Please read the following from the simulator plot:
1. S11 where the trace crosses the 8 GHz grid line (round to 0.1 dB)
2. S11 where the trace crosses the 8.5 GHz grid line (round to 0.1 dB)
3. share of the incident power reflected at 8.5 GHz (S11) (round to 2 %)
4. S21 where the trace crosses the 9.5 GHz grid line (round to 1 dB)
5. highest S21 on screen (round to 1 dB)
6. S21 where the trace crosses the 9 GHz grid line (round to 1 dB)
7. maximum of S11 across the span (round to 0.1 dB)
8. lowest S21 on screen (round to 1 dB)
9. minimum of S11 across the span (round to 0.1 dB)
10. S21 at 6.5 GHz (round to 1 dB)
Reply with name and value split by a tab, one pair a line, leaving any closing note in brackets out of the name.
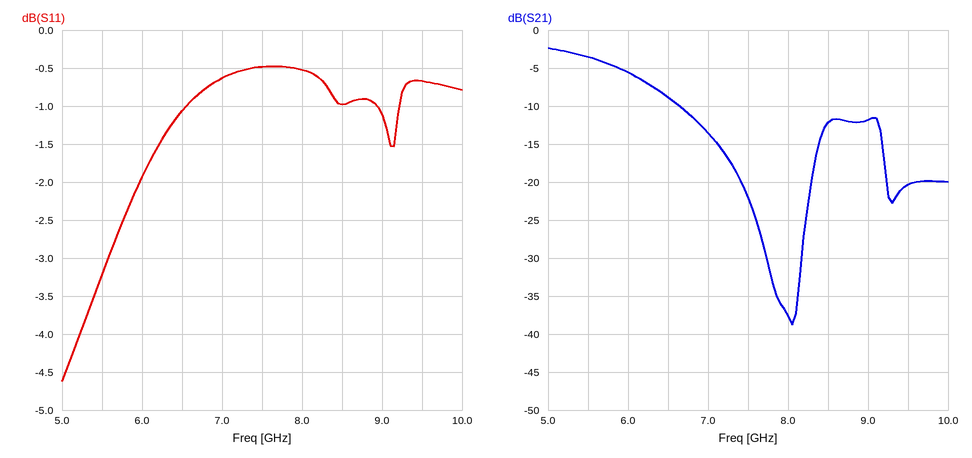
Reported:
S11 where the trace crosses the 8 GHz grid line	-0.5 dB
S11 where the trace crosses the 8.5 GHz grid line	-1.0 dB
share of the incident power reflected at 8.5 GHz (S11)	80 %
S21 where the trace crosses the 9.5 GHz grid line	-20 dB
highest S21 on screen	-2 dB
S21 where the trace crosses the 9 GHz grid line	-12 dB
maximum of S11 across the span	-0.5 dB
lowest S21 on screen	-39 dB
minimum of S11 across the span	-4.6 dB
S21 at 6.5 GHz	-9 dB
